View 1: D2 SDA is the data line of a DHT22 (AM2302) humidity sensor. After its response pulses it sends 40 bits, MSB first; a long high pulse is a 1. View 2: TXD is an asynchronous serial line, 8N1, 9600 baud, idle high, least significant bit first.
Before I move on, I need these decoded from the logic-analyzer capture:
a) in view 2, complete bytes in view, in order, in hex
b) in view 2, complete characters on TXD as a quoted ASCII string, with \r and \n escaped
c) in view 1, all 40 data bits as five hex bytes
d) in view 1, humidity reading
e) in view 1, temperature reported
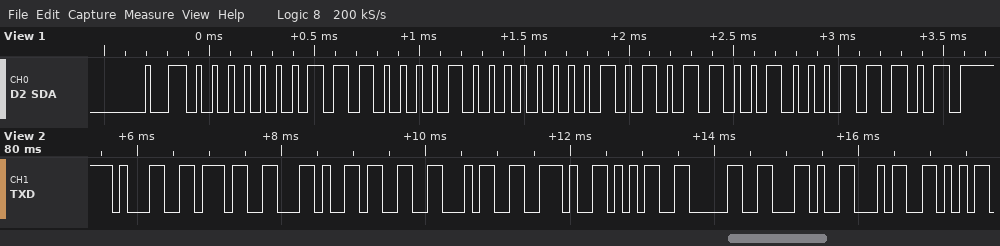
31 37 2C 33 34 2E 35 30 2C 34
"17,34.50,4"
01 C2 01 59 1D
45.0 %
34.5 °C
